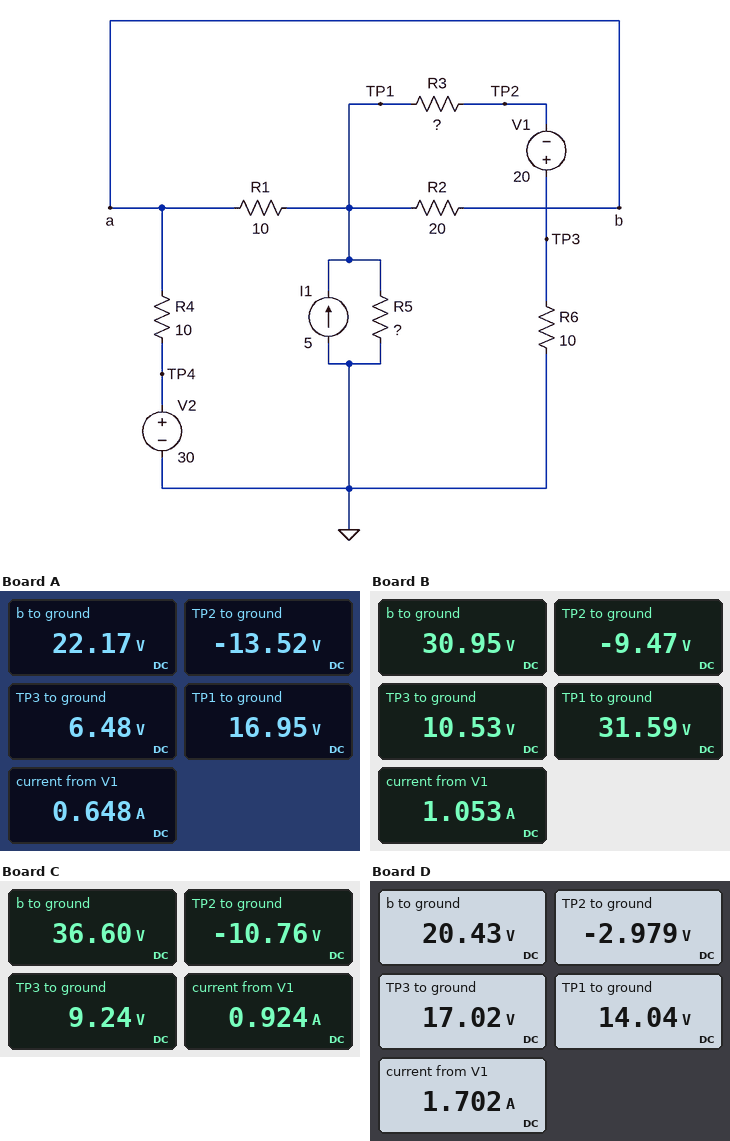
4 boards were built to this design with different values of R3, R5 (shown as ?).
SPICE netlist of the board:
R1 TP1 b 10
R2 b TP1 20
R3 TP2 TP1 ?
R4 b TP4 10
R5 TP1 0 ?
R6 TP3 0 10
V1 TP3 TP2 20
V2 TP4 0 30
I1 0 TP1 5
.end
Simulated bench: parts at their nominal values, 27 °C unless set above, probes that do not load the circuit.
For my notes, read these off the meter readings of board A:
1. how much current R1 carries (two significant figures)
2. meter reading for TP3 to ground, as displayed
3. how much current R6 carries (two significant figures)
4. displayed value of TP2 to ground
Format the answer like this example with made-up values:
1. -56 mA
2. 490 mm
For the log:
1. 520 mA
2. 6.48 V
3. 650 mA
4. -13.52 V
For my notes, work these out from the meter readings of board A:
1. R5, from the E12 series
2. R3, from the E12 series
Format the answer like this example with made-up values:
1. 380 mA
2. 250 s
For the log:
1. 3.3 Ω
2. 47 Ω
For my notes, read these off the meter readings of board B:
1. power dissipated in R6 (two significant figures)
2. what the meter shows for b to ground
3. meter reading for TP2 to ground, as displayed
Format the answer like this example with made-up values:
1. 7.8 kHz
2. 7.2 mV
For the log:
1. 11 W
2. 30.95 V
3. -9.47 V
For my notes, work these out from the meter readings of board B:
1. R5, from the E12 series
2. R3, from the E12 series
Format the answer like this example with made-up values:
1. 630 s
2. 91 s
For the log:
1. 8.2 Ω
2. 39 Ω
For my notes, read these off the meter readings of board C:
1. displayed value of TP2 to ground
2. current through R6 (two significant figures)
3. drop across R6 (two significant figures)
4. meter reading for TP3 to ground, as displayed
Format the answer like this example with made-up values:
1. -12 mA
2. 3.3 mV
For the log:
1. -10.76 V
2. 920 mA
3. 9.2 V
4. 9.24 V
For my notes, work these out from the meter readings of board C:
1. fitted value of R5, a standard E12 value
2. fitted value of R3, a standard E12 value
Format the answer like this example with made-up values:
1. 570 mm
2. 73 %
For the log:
1. 12 Ω
2. 56 Ω
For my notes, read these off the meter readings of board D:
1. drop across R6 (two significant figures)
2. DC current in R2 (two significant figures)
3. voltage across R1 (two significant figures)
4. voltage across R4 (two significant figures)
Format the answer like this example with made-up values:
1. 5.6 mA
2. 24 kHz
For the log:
1. 17 V
2. 320 mA
3. 6.4 V
4. 9.6 V
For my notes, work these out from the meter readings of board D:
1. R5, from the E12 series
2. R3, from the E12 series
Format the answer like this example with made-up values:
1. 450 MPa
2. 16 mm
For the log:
1. 3.3 Ω
2. 10 Ω
